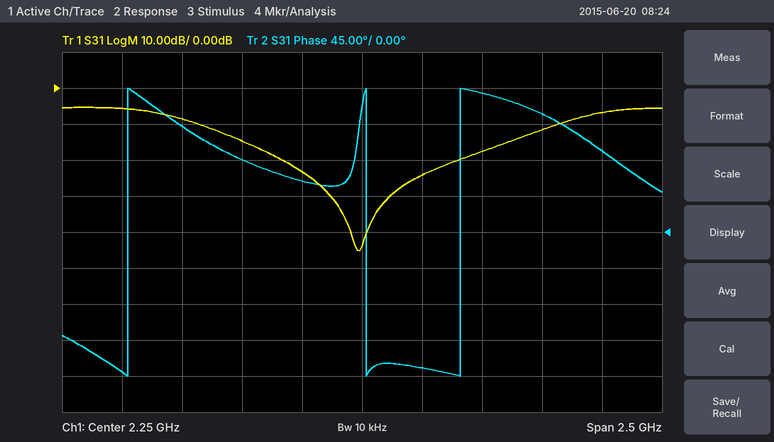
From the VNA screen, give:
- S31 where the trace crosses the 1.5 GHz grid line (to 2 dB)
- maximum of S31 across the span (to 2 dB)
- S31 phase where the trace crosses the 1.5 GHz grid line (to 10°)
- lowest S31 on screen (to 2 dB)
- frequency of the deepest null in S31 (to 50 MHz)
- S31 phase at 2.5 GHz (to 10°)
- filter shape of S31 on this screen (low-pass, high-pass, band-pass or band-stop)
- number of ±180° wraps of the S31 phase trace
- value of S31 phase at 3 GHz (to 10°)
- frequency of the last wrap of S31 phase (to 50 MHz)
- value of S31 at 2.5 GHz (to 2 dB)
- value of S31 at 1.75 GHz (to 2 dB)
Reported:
-8 dB
-6 dB
130°
-46 dB
2.25 GHz
-170°
band-stop
3
150°
2.65 GHz
-24 dB
-14 dB
